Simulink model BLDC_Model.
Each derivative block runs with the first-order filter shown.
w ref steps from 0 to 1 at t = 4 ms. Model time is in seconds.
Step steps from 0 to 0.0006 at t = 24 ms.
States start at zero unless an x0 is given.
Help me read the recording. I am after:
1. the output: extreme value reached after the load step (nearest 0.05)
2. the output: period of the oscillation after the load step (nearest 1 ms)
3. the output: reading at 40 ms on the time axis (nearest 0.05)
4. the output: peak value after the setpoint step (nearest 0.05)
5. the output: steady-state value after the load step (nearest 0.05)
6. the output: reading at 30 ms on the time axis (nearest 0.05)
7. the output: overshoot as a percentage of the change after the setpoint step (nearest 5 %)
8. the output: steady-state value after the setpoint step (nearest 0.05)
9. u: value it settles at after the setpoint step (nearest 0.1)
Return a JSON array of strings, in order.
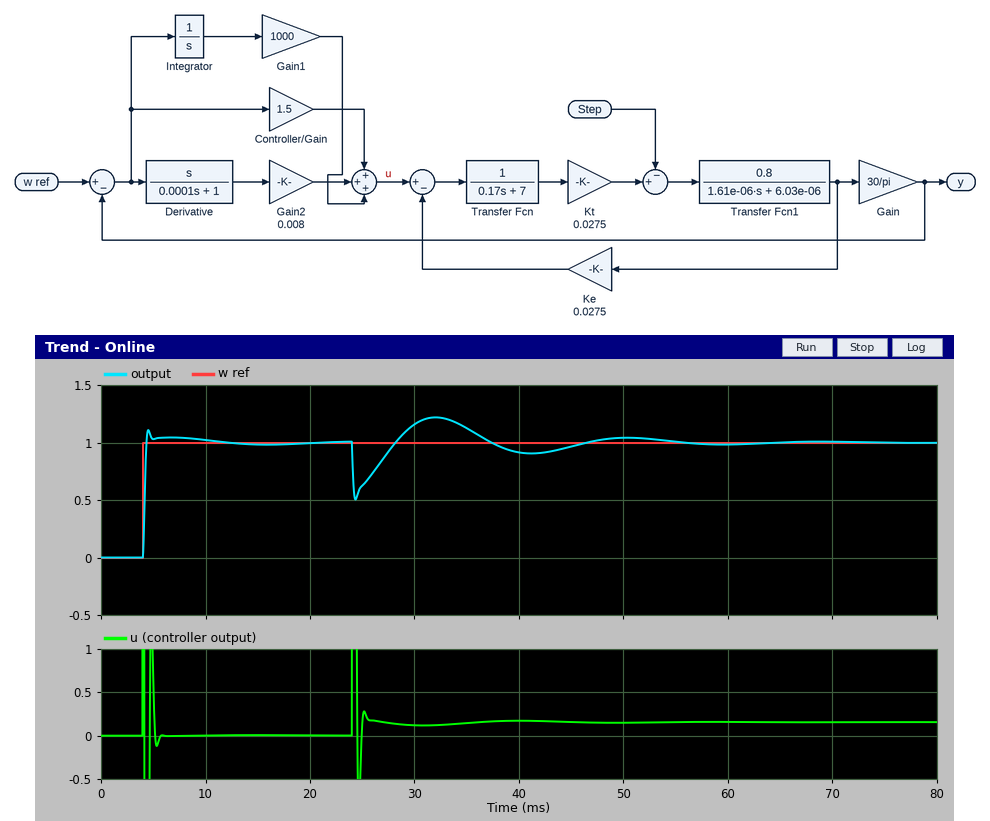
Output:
["0.50", "17 ms", "0.90", "1.10", "1.00", "1.15", "10 %", "1.00", "0.0"]
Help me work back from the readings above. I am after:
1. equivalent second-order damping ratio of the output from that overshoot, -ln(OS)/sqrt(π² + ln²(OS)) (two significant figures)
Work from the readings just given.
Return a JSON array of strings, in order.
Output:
["0.59"]
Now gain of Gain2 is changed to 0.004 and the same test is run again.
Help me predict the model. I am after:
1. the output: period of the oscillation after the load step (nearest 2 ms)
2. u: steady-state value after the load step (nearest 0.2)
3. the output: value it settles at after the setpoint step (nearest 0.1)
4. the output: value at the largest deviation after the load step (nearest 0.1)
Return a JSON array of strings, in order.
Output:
["12 ms", "0.2", "1.0", "0.2"]
